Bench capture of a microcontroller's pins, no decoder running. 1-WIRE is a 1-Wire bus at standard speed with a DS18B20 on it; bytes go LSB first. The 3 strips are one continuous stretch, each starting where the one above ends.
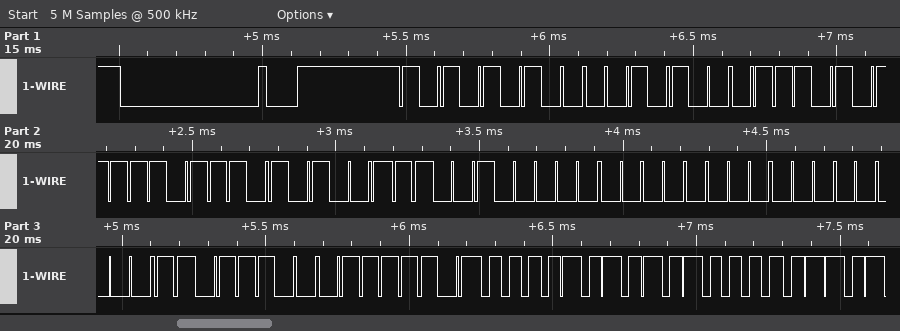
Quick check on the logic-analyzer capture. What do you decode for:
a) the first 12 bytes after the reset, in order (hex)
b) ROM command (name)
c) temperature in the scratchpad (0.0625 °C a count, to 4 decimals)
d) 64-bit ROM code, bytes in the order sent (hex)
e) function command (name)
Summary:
55 28 AE 77 E5 04 00 00 3B BE 50 05
Match ROM
85.0000 °C
28 AE 77 E5 04 00 00 3B
Read Scratchpad
